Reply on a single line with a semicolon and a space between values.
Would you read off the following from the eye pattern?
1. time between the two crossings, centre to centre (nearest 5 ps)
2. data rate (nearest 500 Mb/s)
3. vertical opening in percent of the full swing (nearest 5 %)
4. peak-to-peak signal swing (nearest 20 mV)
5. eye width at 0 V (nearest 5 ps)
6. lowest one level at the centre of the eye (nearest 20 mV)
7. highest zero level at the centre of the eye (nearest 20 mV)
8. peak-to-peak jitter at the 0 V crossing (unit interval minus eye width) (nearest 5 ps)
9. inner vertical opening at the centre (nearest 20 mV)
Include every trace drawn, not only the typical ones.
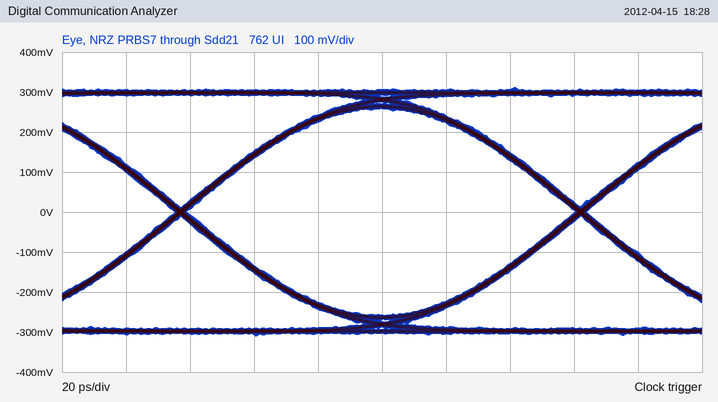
125 ps; 8.0 Gb/s; 85 %; 620 mV; 120 ps; 260 mV; -260 mV; 5 ps; 520 mV
